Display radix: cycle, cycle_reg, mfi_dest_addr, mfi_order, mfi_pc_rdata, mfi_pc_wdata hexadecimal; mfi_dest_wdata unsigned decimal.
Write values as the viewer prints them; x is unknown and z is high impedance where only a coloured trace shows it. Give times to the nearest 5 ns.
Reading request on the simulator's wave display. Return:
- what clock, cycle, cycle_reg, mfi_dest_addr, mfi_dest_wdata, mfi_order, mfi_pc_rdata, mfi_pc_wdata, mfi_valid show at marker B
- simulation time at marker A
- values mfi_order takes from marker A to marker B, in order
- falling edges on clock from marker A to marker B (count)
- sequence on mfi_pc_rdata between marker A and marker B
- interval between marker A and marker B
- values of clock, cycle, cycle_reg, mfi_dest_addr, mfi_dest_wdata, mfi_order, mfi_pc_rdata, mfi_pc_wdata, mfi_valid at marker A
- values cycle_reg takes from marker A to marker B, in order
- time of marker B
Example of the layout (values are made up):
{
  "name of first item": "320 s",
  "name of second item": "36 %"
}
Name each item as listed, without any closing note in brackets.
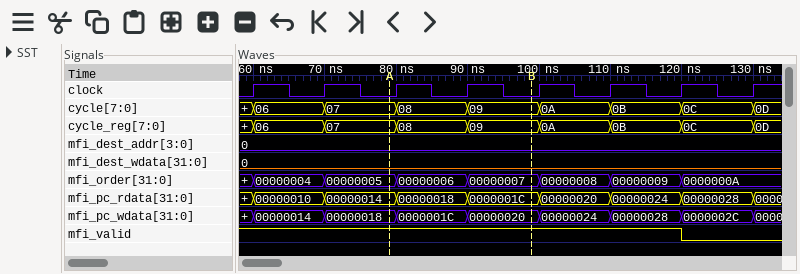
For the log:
{
  "what clock, cycle, cycle_reg, mfi_dest_addr, mfi_dest_wdata, mfi_order, mfi_pc_rdata, mfi_pc_wdata, mfi_valid show at marker B": "clock=0, cycle=09, cycle_reg=09, mfi_dest_addr=0, mfi_dest_wdata=0, mfi_order=00000007, mfi_pc_rdata=0000001C, mfi_pc_wdata=00000020, mfi_valid=1",
  "simulation time at marker A": "80 ns",
  "values mfi_order takes from marker A to marker B, in order": "00000005, 00000006, 00000007",
  "falling edges on clock from marker A to marker B": "2",
  "sequence on mfi_pc_rdata between marker A and marker B": "00000014, 00000018, 0000001C",
  "interval between marker A and marker B": "20 ns",
  "values of clock, cycle, cycle_reg, mfi_dest_addr, mfi_dest_wdata, mfi_order, mfi_pc_rdata, mfi_pc_wdata, mfi_valid at marker A": "clock=0, cycle=07, cycle_reg=07, mfi_dest_addr=0, mfi_dest_wdata=0, mfi_order=00000005, mfi_pc_rdata=00000014, mfi_pc_wdata=00000018, mfi_valid=1",
  "values cycle_reg takes from marker A to marker B, in order": "07, 08, 09",
  "time of marker B": "100 ns"
}
